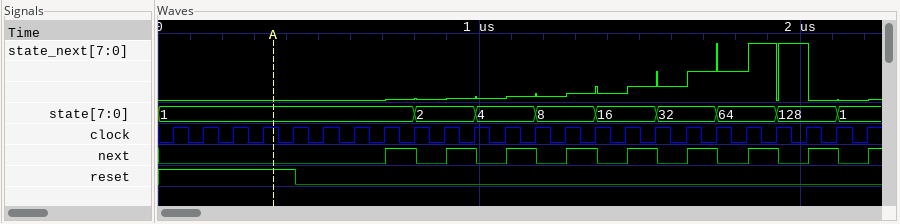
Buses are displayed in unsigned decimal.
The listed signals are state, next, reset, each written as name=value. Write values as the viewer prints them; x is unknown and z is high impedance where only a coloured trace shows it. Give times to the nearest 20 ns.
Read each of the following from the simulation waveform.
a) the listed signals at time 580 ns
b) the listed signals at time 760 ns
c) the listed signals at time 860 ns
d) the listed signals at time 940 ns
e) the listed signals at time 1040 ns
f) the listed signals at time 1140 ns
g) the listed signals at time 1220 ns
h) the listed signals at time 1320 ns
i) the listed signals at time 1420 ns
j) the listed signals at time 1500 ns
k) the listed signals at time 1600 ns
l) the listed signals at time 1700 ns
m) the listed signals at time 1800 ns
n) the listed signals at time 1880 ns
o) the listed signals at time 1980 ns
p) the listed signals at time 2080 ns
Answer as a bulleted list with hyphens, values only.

- state=1, next=0, reset=0
- state=1, next=1, reset=0
- state=2, next=0, reset=0
- state=2, next=1, reset=0
- state=4, next=0, reset=0
- state=4, next=1, reset=0
- state=8, next=0, reset=0
- state=8, next=1, reset=0
- state=16, next=0, reset=0
- state=16, next=1, reset=0
- state=32, next=0, reset=0
- state=32, next=1, reset=0
- state=64, next=0, reset=0
- state=64, next=1, reset=0
- state=128, next=0, reset=0
- state=128, next=1, reset=0
